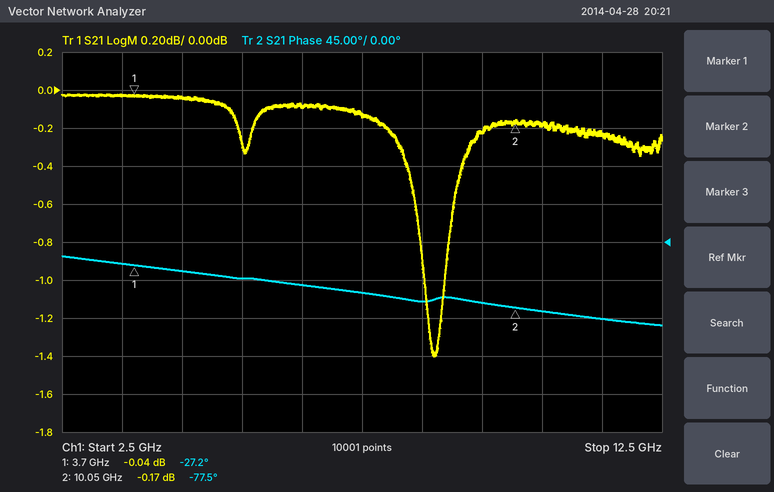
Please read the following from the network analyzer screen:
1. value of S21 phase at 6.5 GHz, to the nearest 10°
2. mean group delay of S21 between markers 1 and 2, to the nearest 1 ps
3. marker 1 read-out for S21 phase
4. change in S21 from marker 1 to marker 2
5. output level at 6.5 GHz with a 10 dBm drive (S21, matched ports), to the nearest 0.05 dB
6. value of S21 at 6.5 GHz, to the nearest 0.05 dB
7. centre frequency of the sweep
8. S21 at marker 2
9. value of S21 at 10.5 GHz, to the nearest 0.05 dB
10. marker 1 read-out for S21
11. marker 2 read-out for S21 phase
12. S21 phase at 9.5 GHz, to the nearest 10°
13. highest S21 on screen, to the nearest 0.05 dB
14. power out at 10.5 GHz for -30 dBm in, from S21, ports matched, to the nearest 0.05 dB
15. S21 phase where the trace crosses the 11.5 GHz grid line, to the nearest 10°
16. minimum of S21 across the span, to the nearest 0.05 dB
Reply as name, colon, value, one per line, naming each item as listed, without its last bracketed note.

value of S21 phase at 6.5 GHz, to the nearest 10°: -50°
mean group delay of S21 between markers 1 and 2, to the nearest 1 ps: 22 ps
marker 1 read-out for S21 phase: -27.2°
change in S21 from marker 1 to marker 2: -0.13 dB
output level at 6.5 GHz with a 10 dBm drive (S21, matched ports), to the nearest 0.05 dB: 9.90 dBm
value of S21 at 6.5 GHz, to the nearest 0.05 dB: -0.10 dB
centre frequency of the sweep: 7.5 GHz
S21 at marker 2: -0.17 dB
value of S21 at 10.5 GHz, to the nearest 0.05 dB: -0.20 dB
marker 1 read-out for S21: -0.04 dB
marker 2 read-out for S21 phase: -77.5°
S21 phase at 9.5 GHz, to the nearest 10°: -70°
highest S21 on screen, to the nearest 0.05 dB: 0.00 dB
power out at 10.5 GHz for -30 dBm in, from S21, ports matched, to the nearest 0.05 dB: -30.20 dBm
S21 phase where the trace crosses the 11.5 GHz grid line, to the nearest 10°: -90°
minimum of S21 across the span, to the nearest 0.05 dB: -1.40 dB
